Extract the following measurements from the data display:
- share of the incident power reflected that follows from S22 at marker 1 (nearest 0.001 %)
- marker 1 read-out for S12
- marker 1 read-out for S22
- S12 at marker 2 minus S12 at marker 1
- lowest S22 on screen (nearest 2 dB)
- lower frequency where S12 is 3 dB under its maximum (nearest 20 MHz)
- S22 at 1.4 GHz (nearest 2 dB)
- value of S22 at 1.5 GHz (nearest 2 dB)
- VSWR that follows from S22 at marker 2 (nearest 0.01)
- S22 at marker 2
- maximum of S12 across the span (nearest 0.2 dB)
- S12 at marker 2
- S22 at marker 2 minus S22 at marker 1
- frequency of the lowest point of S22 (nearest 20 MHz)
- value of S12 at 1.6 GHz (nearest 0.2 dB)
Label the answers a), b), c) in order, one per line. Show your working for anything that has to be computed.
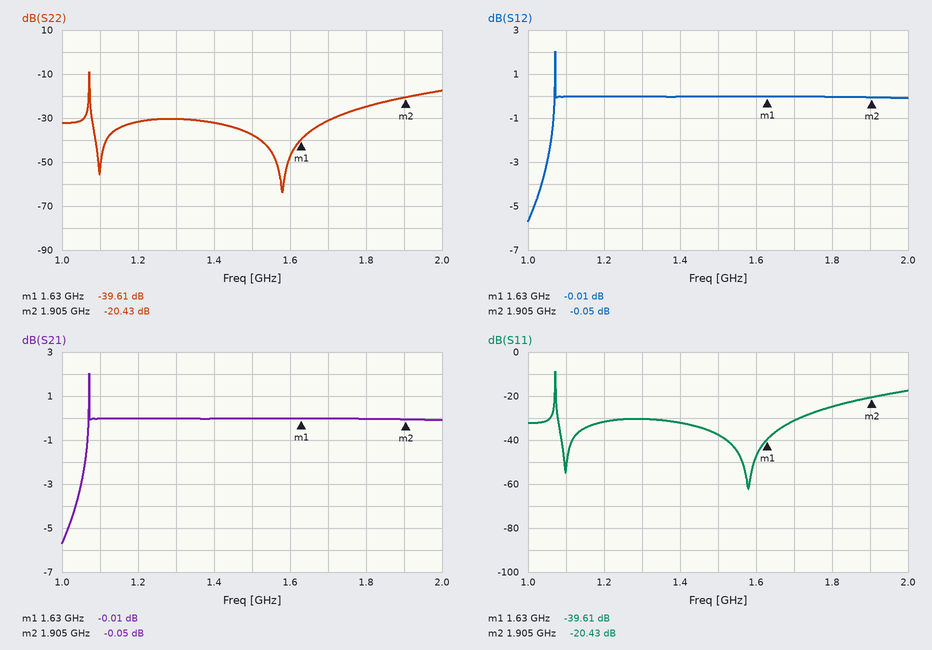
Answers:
a) 10^(-39.61/10) ≈ 0.011 %
b) -0.01 dB
c) -39.61 dB
d) -0.05 − (-0.01) = -0.04 dB
e) -64 dB
f) 1.06 GHz
g) -32 dB
h) -38 dB
i) (1 + 0.0952)/(1 − 0.0952) ≈ 1.21
j) -20.43 dB
k) 2.0 dB
l) -0.05 dB
m) -20.43 − (-39.61) = 19.18 dB
n) 1.58 GHz
o) 0.0 dB
